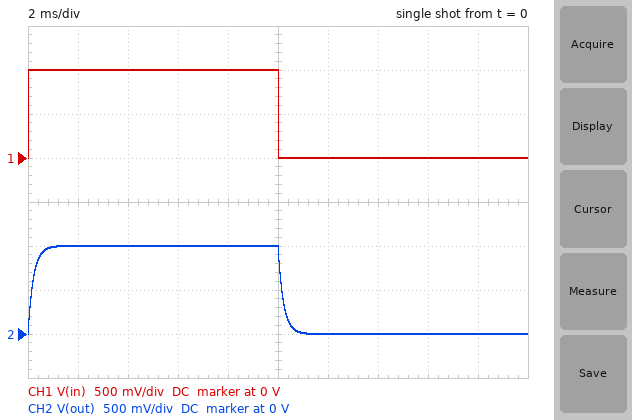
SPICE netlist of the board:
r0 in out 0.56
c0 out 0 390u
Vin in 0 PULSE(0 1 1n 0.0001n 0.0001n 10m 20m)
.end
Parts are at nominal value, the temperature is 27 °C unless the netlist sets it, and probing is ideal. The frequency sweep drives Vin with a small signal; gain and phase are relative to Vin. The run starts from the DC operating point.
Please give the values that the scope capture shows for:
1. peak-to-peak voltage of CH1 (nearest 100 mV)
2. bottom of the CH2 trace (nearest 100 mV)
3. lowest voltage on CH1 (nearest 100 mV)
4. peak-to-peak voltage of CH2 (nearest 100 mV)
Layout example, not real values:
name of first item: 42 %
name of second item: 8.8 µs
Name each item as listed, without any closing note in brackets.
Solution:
peak-to-peak voltage of CH1: 1.0 V
bottom of the CH2 trace: 0 V
lowest voltage on CH1: 0 V
peak-to-peak voltage of CH2: 1.0 V
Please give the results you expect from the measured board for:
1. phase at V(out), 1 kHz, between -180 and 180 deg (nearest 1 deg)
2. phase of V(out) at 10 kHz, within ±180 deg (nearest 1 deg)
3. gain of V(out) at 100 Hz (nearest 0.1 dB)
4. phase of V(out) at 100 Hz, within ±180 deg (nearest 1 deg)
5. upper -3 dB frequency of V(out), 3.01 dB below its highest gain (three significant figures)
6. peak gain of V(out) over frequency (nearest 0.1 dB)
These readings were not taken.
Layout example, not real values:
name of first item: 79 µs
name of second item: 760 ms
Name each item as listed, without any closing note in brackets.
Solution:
phase at V(out), 1 kHz, between -180 and 180 deg: -54 deg
phase of V(out) at 10 kHz, within ±180 deg: -86 deg
gain of V(out) at 100 Hz: -0.1 dB
phase of V(out) at 100 Hz, within ±180 deg: -8 deg
upper -3 dB frequency of V(out), 3.01 dB below its highest gain: 729 Hz
peak gain of V(out) over frequency: 0 dB
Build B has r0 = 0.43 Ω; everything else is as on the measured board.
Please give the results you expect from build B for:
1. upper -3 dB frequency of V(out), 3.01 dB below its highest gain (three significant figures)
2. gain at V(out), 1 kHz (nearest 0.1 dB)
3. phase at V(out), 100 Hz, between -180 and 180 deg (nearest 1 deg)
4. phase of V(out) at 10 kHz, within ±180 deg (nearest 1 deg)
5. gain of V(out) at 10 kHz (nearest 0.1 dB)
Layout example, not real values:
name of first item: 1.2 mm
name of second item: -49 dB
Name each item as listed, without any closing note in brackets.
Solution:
upper -3 dB frequency of V(out), 3.01 dB below its highest gain: 949 Hz
gain at V(out), 1 kHz: -3.2 dB
phase at V(out), 100 Hz, between -180 and 180 deg: -6 deg
phase of V(out) at 10 kHz, within ±180 deg: -85 deg
gain of V(out) at 10 kHz: -20.5 dB
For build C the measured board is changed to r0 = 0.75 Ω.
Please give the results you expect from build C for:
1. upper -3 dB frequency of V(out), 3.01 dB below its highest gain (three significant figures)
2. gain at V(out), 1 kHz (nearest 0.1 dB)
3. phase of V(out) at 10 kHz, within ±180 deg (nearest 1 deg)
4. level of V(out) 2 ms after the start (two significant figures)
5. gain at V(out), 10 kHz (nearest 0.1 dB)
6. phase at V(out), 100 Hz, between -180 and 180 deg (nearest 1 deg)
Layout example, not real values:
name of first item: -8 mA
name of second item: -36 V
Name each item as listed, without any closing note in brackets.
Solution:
upper -3 dB frequency of V(out), 3.01 dB below its highest gain: 544 Hz
gain at V(out), 1 kHz: -6.4 dB
phase of V(out) at 10 kHz, within ±180 deg: -87 deg
level of V(out) 2 ms after the start: 1.0 V
gain at V(out), 10 kHz: -25.3 dB
phase at V(out), 100 Hz, between -180 and 180 deg: -10 deg
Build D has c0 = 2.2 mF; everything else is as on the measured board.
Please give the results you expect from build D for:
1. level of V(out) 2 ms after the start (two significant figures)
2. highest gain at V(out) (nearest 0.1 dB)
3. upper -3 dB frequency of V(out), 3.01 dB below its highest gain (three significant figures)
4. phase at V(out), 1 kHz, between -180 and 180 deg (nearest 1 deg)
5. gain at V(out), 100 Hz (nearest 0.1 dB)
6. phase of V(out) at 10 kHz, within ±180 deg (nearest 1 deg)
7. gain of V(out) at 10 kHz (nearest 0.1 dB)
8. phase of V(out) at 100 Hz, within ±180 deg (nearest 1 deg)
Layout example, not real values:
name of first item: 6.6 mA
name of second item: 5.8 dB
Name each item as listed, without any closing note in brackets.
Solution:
level of V(out) 2 ms after the start: 800 mV
highest gain at V(out): 0 dB
upper -3 dB frequency of V(out), 3.01 dB below its highest gain: 129 Hz
phase at V(out), 1 kHz, between -180 and 180 deg: -83 deg
gain at V(out), 100 Hz: -2.0 dB
phase of V(out) at 10 kHz, within ±180 deg: -89 deg
gain of V(out) at 10 kHz: -37.8 dB
phase of V(out) at 100 Hz, within ±180 deg: -38 deg
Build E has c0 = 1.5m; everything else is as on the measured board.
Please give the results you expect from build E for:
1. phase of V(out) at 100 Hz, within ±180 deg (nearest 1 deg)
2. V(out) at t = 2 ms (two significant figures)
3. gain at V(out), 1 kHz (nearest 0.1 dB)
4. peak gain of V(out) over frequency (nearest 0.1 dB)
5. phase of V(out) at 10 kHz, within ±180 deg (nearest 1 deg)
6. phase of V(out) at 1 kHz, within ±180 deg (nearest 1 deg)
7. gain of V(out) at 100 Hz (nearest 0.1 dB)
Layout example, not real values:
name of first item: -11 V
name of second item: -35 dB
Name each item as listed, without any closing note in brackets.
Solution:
phase of V(out) at 100 Hz, within ±180 deg: -28 deg
V(out) at t = 2 ms: 910 mV
gain at V(out), 1 kHz: -14.6 dB
peak gain of V(out) over frequency: 0 dB
phase of V(out) at 10 kHz, within ±180 deg: -89 deg
phase of V(out) at 1 kHz, within ±180 deg: -79 deg
gain of V(out) at 100 Hz: -1.1 dB
